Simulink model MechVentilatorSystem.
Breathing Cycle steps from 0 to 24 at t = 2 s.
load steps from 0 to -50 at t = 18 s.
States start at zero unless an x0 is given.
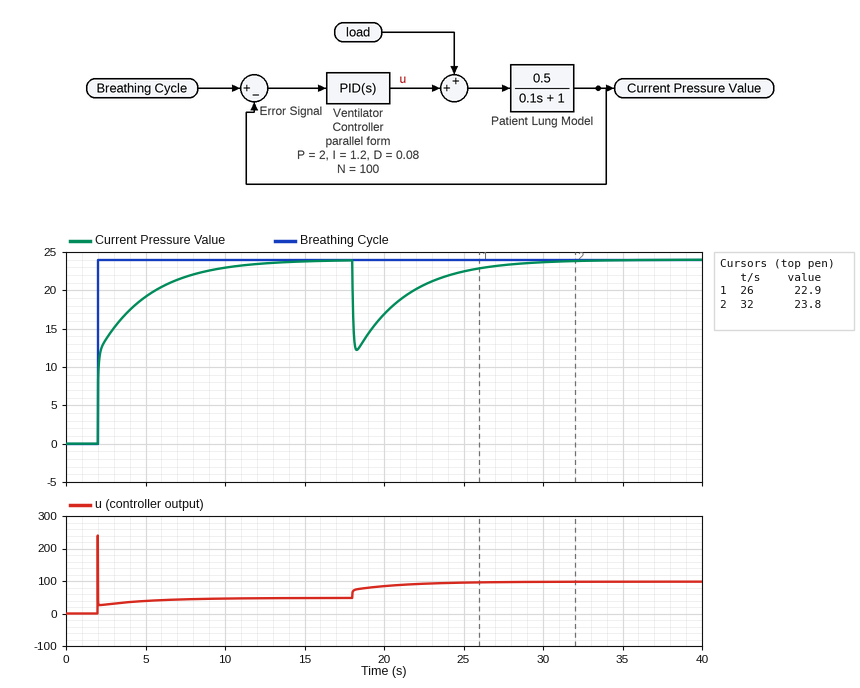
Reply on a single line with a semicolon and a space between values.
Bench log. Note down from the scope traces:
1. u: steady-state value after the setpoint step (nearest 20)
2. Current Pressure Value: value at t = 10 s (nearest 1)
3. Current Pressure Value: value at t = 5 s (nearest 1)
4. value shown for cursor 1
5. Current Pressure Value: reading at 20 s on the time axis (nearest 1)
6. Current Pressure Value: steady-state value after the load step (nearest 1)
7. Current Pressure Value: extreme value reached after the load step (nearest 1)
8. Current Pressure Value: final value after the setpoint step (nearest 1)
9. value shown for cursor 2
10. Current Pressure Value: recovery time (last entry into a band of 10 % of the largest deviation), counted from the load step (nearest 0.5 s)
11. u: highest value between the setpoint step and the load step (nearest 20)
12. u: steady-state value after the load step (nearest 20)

40; 23; 19; 22.9; 17; 24; 12; 24; 23.8; 8.0 s; 240; 100
